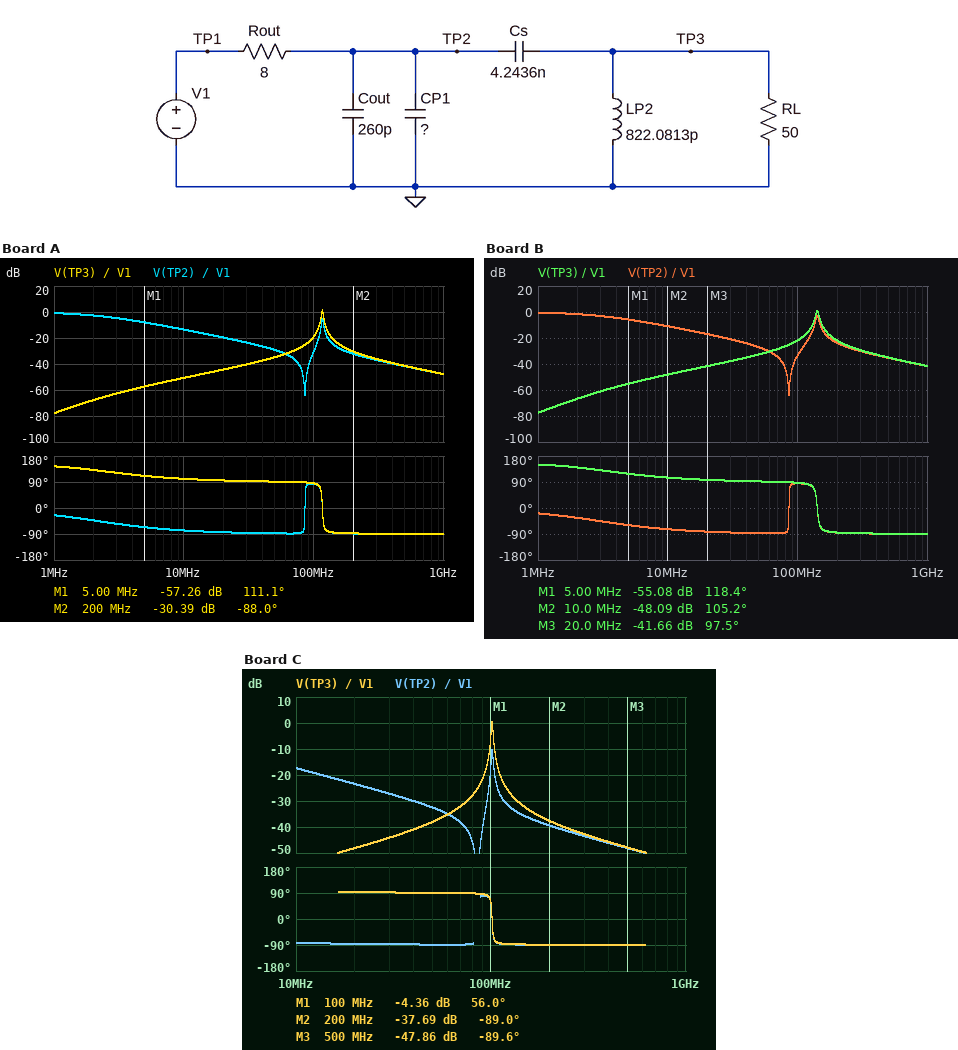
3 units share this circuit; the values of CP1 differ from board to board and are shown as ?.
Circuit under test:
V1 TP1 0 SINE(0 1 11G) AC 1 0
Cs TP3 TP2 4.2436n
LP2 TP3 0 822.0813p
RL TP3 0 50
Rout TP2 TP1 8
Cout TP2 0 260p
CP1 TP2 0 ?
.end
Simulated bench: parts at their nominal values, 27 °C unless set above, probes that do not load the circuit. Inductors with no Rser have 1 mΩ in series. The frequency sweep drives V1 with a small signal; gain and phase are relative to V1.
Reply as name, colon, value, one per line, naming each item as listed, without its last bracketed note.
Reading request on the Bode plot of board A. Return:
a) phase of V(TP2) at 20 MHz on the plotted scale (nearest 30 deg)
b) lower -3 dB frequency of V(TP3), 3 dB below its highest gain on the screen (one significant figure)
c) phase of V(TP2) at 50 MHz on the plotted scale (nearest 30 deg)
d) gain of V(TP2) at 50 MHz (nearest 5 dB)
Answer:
phase of V(TP2) at 20 MHz on the plotted scale: -90 deg
lower -3 dB frequency of V(TP3), 3 dB below its highest gain on the screen: 100 MHz
phase of V(TP2) at 50 MHz on the plotted scale: -90 deg
gain of V(TP2) at 50 MHz: -30 dB
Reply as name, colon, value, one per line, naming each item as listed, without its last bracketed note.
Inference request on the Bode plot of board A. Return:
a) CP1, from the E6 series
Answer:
CP1, from the E6 series: 4.7 nF
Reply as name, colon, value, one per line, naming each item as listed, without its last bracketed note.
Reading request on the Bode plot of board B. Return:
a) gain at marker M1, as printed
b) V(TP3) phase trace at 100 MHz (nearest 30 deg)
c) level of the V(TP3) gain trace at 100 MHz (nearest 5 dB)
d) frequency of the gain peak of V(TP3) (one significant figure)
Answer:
gain at marker M1, as printed: -55.08 dB
V(TP3) phase trace at 100 MHz: 90 deg
level of the V(TP3) gain trace at 100 MHz: -20 dB
frequency of the gain peak of V(TP3): 100 MHz
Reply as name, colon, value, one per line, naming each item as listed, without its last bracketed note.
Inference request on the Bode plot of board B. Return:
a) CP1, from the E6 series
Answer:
CP1, from the E6 series: 2.2 nF
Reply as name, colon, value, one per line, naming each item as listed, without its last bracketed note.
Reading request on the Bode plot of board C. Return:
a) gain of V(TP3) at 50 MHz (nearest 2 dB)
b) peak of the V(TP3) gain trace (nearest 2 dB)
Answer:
gain of V(TP3) at 50 MHz: -38 dB
peak of the V(TP3) gain trace: 0 dB
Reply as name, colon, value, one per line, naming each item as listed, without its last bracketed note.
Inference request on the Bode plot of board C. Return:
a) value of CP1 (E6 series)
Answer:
value of CP1: 10 nF
